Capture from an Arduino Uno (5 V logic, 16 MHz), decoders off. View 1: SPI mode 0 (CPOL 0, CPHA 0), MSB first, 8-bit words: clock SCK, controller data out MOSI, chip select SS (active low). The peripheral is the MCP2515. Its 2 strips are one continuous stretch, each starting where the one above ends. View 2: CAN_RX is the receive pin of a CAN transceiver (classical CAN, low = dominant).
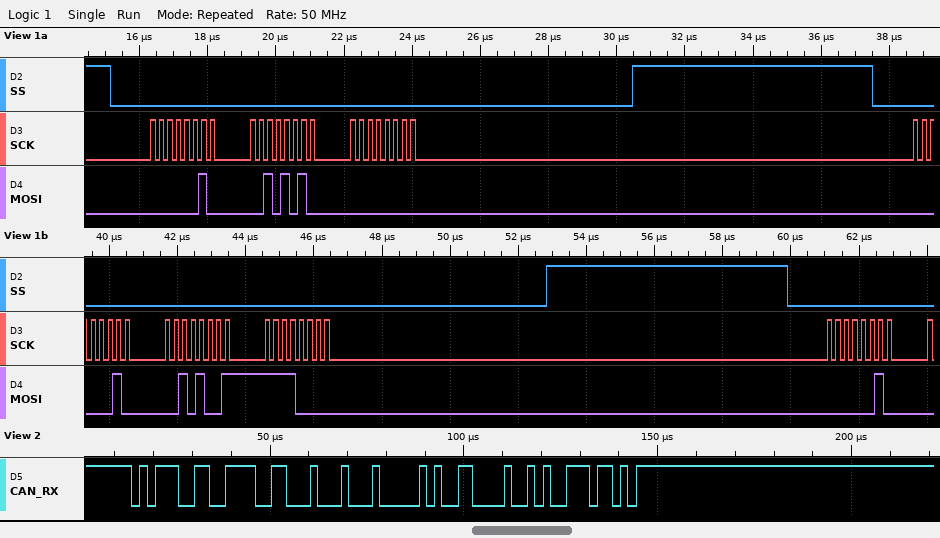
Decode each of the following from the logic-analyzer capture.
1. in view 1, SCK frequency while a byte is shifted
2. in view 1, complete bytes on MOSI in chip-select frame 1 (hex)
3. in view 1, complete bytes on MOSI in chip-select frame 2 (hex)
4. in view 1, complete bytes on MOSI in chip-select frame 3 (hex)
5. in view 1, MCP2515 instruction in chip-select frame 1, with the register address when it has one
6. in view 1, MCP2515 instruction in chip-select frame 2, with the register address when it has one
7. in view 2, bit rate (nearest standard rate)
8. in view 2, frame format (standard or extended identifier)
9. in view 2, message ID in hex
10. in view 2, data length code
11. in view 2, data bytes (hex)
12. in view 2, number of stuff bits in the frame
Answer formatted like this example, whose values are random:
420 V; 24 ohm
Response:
4 MHz; 02 2A 00; 02 29 F0; 02; WRITE 0x2A; WRITE 0x29; 500 kbit/s; extended; 0x17333111; 1; 30; 1
